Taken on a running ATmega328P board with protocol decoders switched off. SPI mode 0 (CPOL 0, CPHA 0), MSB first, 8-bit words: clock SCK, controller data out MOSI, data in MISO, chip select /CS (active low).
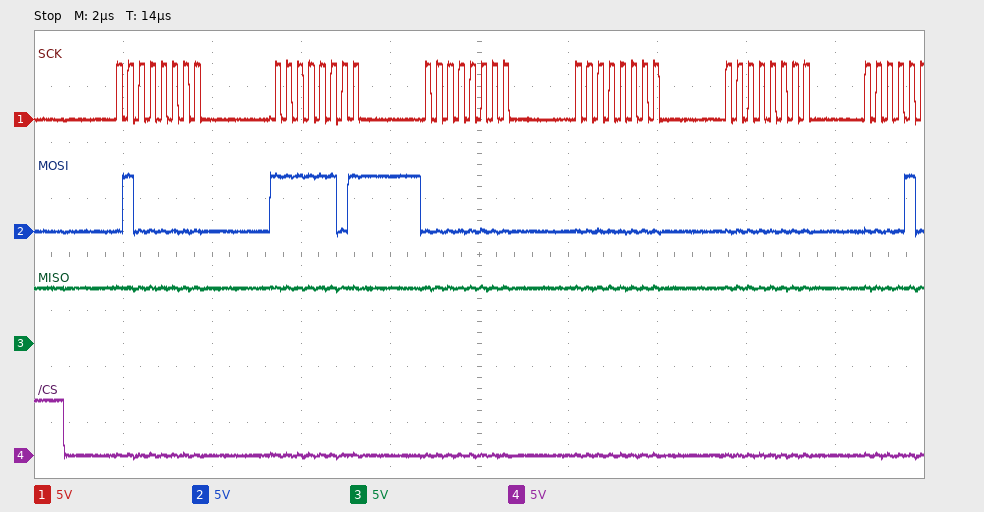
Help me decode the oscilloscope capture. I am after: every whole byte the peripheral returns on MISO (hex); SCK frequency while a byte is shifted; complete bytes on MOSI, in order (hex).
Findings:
0xFF 0xFF 0xFF 0xFF 0xFF
4 MHz
0x40 0xFD 0x00 0x00 0x00
